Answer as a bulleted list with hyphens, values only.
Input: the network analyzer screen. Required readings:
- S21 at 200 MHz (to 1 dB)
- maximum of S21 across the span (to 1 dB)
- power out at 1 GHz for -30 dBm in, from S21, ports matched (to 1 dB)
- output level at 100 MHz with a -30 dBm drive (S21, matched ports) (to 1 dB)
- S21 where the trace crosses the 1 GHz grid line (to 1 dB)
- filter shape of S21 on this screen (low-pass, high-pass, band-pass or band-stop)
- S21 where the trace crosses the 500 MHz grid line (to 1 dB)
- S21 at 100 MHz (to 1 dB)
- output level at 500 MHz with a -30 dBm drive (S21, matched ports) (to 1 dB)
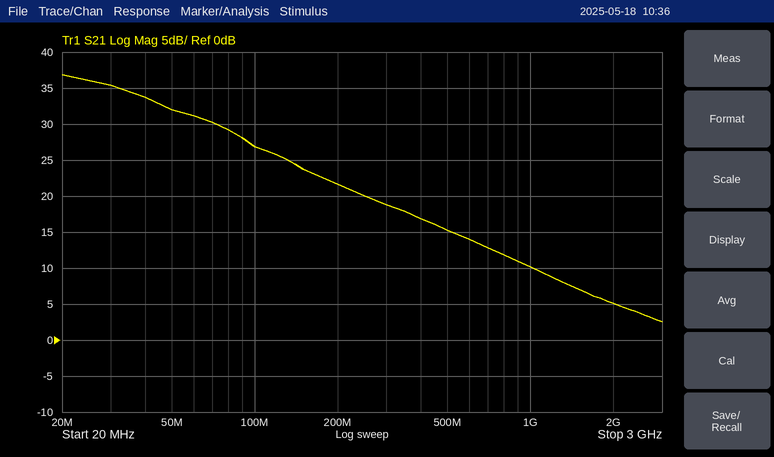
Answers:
- 22 dB
- 37 dB
- -20 dBm
- -3 dBm
- 10 dB
- low-pass
- 15 dB
- 27 dB
- -15 dBm
